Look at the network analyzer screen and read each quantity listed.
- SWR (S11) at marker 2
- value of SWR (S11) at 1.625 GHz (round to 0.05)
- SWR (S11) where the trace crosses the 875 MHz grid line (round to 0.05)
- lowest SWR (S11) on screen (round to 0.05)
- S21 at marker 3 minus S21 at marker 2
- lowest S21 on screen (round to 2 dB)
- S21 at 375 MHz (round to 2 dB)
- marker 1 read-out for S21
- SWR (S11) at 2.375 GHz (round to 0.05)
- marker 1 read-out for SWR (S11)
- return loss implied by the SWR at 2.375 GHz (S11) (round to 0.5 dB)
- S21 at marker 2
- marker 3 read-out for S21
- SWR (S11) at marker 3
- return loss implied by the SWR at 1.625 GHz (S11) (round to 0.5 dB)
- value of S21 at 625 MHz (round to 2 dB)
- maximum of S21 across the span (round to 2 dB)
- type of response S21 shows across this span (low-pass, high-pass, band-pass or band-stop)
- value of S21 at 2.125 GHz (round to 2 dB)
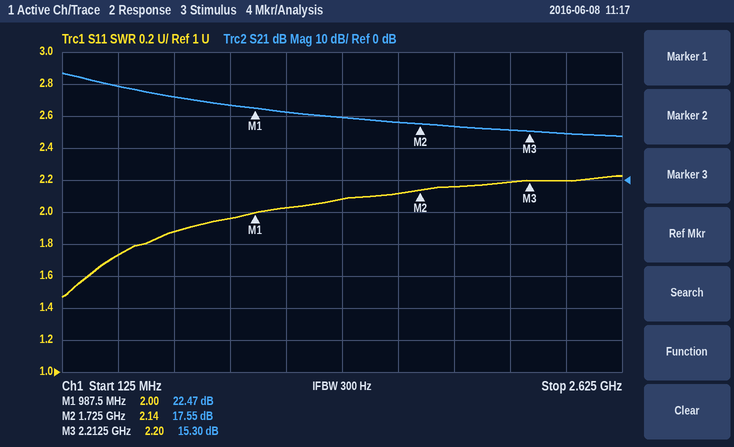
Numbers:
2.14
2.10
1.95
1.45
-2.25 dB
14 dB
30 dB
22.47 dB
2.20
2.00
8.5 dB
17.55 dB
15.30 dB
2.20
9.0 dB
26 dB
34 dB
low-pass
16 dB
